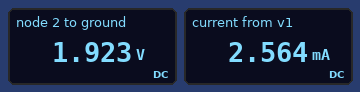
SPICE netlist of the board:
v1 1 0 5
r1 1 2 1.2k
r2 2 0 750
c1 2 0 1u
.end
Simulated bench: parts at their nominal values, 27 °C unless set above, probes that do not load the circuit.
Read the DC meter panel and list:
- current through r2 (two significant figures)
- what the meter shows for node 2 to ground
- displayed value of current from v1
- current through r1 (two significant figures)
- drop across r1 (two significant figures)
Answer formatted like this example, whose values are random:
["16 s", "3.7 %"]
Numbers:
["2.6 mA", "1.923 V", "2.564 mA", "2.6 mA", "3.1 V"]
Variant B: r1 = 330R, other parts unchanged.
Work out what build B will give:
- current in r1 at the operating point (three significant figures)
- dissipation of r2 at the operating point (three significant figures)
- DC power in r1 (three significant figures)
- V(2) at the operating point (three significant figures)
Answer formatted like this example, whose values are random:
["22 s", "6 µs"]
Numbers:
["4.63 mA", "16.1 mW", "7.07 mW", "3.47 V"]
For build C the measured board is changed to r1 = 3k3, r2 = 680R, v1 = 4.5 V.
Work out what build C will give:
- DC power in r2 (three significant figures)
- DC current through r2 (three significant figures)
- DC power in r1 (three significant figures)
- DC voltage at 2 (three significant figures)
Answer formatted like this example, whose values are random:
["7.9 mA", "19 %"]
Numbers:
["869 µW", "1.13 mA", "4.22 mW", "769 mV"]
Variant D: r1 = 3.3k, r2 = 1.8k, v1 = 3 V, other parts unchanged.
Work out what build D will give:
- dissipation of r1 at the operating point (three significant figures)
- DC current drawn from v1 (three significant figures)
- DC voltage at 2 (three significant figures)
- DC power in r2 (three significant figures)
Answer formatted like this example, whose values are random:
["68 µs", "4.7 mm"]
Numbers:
["1.14 mW", "588 µA", "1.06 V", "623 µW"]
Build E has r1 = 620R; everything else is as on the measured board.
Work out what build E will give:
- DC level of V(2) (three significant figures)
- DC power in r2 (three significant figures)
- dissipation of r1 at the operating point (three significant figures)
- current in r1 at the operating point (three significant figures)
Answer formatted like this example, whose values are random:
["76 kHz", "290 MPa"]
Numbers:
["2.74 V", "9.99 mW", "8.26 mW", "3.65 mA"]
